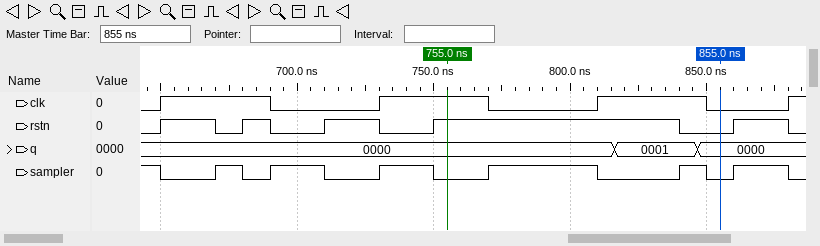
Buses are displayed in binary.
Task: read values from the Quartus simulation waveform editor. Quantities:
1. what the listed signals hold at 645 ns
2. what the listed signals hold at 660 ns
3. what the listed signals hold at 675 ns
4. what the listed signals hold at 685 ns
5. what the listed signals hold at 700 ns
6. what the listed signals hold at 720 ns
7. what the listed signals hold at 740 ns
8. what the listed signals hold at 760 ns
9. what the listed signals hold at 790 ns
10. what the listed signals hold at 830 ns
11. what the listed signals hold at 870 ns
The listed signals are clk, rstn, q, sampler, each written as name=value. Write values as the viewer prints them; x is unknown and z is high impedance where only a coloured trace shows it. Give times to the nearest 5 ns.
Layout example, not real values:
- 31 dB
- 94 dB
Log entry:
- clk=0, rstn=0, q=0000, sampler=1
- clk=1, rstn=1, q=0000, sampler=0
- clk=1, rstn=0, q=0000, sampler=1
- clk=1, rstn=1, q=0000, sampler=0
- clk=0, rstn=0, q=0000, sampler=1
- clk=0, rstn=1, q=0000, sampler=0
- clk=1, rstn=0, q=0000, sampler=1
- clk=1, rstn=1, q=0000, sampler=0
- clk=0, rstn=1, q=0000, sampler=1
- clk=1, rstn=1, q=0001, sampler=0
- clk=0, rstn=1, q=0000, sampler=1
